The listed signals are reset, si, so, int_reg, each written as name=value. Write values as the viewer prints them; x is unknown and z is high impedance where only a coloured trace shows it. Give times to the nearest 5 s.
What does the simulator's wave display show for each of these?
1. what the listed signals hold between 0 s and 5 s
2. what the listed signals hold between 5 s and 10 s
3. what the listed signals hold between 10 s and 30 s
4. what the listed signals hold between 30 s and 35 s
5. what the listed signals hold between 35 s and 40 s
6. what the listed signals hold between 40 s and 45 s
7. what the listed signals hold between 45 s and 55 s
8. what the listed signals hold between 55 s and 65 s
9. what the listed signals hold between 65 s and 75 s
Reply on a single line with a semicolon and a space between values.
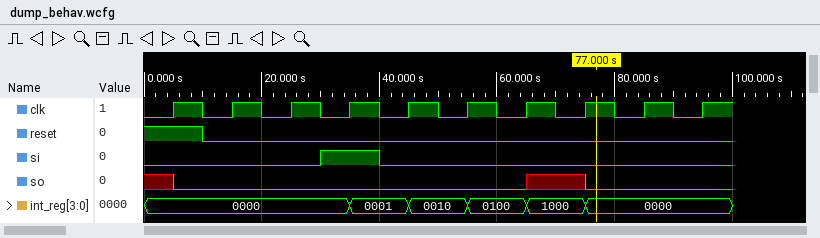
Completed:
reset=1, si=0, so=x, int_reg=0000; reset=1, si=0, so=0, int_reg=0000; reset=0, si=0, so=0, int_reg=0000; reset=0, si=1, so=0, int_reg=0000; reset=0, si=1, so=0, int_reg=0001; reset=0, si=0, so=0, int_reg=0001; reset=0, si=0, so=0, int_reg=0010; reset=0, si=0, so=0, int_reg=0100; reset=0, si=0, so=x, int_reg=1000
